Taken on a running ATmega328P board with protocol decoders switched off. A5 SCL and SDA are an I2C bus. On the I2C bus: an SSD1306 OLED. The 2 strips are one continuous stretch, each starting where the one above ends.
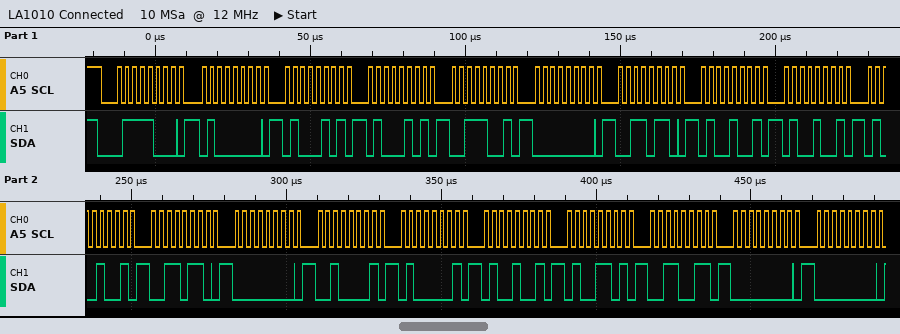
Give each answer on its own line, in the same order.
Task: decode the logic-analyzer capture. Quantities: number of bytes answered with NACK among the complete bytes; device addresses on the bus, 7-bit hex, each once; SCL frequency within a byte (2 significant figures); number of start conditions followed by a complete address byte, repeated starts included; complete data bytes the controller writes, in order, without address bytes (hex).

0
0x3C
400 kHz
1
40 45 45 39 00 36 49 49 49 36 00 21 41 49 4D 33 00 00
